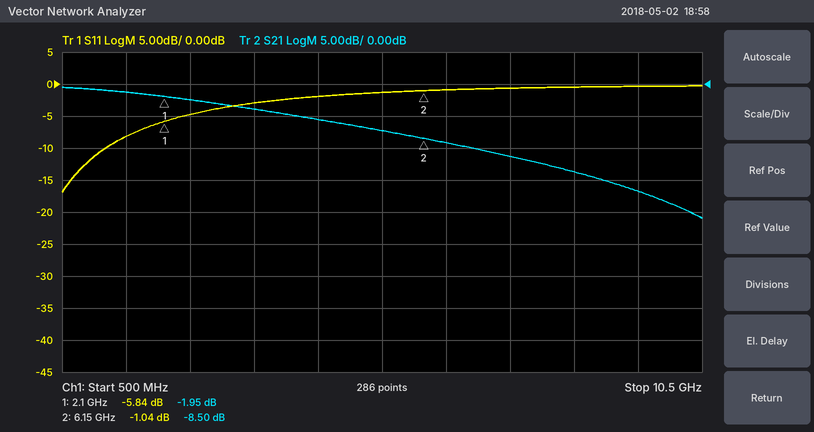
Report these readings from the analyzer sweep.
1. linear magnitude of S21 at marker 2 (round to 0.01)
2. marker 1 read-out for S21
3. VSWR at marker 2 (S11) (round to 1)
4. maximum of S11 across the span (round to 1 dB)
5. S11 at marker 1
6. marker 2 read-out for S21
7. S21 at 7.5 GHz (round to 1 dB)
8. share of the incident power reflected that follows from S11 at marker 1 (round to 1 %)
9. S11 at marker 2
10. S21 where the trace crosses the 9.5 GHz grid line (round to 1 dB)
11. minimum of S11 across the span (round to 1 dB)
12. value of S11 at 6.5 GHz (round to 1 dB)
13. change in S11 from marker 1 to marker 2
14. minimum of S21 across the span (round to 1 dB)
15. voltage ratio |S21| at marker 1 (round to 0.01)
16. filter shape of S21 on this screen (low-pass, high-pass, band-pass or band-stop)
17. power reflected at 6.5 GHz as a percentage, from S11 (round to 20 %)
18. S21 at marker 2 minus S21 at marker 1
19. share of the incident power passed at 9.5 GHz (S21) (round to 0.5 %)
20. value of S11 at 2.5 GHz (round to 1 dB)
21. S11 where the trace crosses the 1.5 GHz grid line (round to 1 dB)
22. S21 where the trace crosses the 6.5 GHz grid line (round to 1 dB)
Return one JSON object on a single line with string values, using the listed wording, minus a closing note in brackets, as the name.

{"linear magnitude of S21 at marker 2": "0.38", "marker 1 read-out for S21": "-1.95 dB", "VSWR at marker 2 (S11)": "17", "maximum of S11 across the span": "0 dB", "S11 at marker 1": "-5.84 dB", "marker 2 read-out for S21": "-8.50 dB", "S21 at 7.5 GHz": "-11 dB", "share of the incident power reflected that follows from S11 at marker 1": "26 %", "S11 at marker 2": "-1.04 dB", "S21 where the trace crosses the 9.5 GHz grid line": "-17 dB", "minimum of S11 across the span": "-17 dB", "value of S11 at 6.5 GHz": "-1 dB", "change in S11 from marker 1 to marker 2": "4.80 dB", "minimum of S21 across the span": "-21 dB", "voltage ratio |S21| at marker 1": "0.80", "filter shape of S21 on this screen": "low-pass", "power reflected at 6.5 GHz as a percentage, from S11": "80 %", "S21 at marker 2 minus S21 at marker 1": "-6.55 dB", "share of the incident power passed at 9.5 GHz (S21)": "2.0 %", "value of S11 at 2.5 GHz": "-5 dB", "S11 where the trace crosses the 1.5 GHz grid line": "-8 dB", "S21 where the trace crosses the 6.5 GHz grid line": "-9 dB"}
